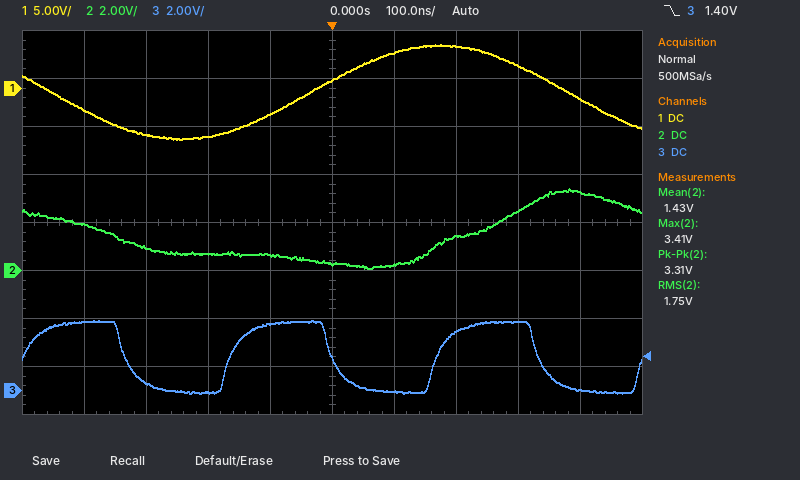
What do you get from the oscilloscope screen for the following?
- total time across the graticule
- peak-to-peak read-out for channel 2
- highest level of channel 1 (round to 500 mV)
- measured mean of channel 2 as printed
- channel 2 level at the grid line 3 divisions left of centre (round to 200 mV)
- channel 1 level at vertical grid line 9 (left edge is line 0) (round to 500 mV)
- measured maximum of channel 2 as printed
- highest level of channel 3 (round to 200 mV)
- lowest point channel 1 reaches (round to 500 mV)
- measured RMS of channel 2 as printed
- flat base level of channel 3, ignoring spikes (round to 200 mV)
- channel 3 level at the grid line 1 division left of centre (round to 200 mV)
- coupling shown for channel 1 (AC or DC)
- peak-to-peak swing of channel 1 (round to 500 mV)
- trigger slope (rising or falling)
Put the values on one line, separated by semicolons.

1 µs; 3.31 V; 4.5 V; 1.43 V; 1.0 V; -1.0 V; 3.41 V; 3.0 V; -5.5 V; 1.75 V; 0.0 V; 2.8 V; DC; 10.0 V; falling
